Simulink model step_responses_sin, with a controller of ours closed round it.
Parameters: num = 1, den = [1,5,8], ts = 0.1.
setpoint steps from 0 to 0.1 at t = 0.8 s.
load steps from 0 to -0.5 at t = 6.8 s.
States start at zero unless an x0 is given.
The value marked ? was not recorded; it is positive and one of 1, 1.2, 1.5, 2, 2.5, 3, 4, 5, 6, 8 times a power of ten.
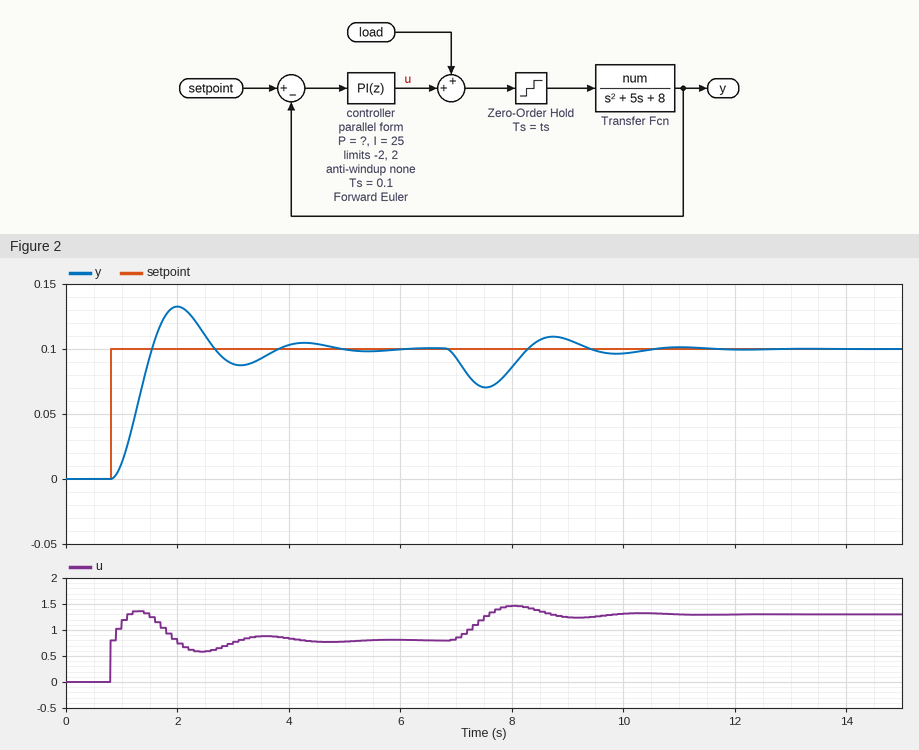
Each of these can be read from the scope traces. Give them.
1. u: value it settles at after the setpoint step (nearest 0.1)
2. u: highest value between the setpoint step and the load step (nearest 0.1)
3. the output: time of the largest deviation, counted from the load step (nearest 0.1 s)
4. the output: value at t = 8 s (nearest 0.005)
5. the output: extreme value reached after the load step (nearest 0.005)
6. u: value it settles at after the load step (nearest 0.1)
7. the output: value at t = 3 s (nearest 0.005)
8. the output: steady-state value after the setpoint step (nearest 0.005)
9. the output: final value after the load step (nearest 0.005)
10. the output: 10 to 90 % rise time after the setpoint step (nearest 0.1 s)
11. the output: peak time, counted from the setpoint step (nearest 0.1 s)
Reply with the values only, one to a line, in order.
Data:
0.8
1.4
0.7 s
0.085
0.070
1.3
0.090
0.100
0.100
0.5 s
1.2 s
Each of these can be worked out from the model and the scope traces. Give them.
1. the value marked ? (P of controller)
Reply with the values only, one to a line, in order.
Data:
8
